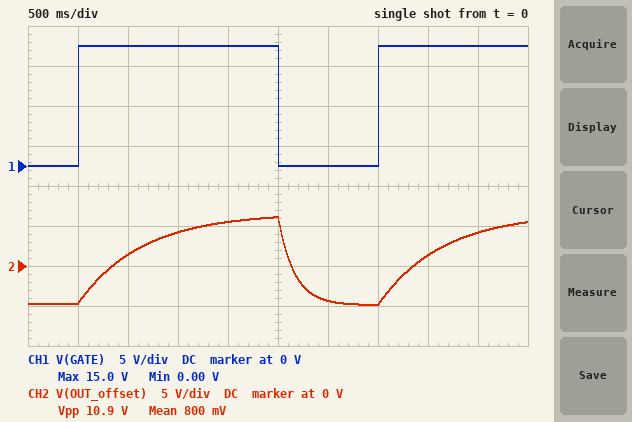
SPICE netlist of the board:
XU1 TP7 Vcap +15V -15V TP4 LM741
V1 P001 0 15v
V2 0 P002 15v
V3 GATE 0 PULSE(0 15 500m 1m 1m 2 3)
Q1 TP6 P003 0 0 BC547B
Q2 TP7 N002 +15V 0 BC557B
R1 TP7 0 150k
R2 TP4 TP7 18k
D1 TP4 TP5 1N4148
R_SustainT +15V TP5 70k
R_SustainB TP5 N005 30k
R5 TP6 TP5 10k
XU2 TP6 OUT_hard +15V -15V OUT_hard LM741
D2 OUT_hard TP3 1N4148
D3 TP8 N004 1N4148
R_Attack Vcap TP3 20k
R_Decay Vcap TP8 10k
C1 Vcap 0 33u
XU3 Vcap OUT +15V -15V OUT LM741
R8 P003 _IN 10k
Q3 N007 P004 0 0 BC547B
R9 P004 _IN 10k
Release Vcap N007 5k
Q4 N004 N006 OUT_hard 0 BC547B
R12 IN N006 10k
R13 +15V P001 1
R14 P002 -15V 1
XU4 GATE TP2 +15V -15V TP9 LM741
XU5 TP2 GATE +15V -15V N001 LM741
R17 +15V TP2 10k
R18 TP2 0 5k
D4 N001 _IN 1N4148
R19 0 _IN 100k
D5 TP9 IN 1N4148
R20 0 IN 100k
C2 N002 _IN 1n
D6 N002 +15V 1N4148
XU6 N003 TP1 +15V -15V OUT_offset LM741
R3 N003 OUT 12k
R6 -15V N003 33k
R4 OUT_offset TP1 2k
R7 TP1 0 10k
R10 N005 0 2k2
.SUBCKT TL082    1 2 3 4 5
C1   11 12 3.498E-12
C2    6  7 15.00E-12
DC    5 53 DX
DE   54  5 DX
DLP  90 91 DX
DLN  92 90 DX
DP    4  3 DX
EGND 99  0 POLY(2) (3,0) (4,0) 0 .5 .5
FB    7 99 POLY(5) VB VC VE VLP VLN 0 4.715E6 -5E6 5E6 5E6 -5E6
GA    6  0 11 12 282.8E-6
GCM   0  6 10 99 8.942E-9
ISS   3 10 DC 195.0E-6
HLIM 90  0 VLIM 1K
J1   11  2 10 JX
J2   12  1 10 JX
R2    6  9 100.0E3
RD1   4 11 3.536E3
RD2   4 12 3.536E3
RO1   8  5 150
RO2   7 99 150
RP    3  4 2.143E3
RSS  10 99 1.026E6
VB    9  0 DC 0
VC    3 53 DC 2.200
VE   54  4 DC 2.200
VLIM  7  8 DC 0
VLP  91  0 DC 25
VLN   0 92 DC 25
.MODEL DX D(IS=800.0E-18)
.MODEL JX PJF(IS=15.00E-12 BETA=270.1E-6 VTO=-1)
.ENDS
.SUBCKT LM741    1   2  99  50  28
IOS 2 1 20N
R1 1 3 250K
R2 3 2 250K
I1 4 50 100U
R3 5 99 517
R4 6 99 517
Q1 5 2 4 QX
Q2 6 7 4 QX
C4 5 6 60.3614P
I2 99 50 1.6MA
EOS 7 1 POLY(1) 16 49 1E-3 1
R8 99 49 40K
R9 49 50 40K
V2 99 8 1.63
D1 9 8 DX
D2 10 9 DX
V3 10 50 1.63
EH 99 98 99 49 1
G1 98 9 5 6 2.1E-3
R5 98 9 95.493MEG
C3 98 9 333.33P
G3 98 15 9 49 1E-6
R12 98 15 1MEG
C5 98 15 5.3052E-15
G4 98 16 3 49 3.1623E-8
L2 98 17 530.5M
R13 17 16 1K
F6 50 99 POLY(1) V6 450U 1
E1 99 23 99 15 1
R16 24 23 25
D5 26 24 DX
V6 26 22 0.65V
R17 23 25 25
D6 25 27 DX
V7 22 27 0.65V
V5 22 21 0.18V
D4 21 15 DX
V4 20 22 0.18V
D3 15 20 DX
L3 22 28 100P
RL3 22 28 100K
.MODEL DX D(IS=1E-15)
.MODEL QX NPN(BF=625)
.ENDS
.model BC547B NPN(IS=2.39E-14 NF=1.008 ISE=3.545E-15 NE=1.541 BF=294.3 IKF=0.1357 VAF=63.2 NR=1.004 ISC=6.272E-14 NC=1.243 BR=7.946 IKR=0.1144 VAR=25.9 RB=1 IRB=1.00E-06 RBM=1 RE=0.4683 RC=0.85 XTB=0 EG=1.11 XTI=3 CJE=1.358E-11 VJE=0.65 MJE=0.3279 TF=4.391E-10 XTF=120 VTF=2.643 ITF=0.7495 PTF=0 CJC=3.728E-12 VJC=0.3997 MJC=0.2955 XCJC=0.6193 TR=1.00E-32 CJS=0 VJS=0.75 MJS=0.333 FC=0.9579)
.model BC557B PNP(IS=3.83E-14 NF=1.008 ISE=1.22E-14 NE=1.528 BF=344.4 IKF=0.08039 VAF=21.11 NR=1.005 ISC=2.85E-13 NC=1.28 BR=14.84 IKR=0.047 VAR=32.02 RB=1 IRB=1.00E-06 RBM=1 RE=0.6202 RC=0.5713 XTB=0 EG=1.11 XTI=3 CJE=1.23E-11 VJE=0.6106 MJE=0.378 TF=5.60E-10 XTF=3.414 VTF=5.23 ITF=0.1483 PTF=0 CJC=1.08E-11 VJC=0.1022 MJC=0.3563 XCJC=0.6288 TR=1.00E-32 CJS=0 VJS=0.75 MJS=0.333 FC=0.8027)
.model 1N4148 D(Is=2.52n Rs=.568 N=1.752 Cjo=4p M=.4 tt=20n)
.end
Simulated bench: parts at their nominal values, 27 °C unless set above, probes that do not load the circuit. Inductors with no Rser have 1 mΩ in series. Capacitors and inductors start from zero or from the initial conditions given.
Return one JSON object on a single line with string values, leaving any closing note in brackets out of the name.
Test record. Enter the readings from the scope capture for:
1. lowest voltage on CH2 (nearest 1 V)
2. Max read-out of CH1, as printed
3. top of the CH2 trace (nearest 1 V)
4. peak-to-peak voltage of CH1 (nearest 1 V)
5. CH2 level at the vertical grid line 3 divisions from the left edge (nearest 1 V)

{"lowest voltage on CH2": "-5 V", "Max read-out of CH1, as printed": "15.0 V", "top of the CH2 trace": "6 V", "peak-to-peak voltage of CH1": "15 V", "CH2 level at the vertical grid line 3 divisions from the left edge": "4 V"}
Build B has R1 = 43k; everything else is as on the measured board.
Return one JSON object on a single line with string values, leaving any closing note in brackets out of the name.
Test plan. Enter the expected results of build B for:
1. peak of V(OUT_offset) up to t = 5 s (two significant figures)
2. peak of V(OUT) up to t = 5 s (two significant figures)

{"peak of V(OUT_offset) up to t = 5 s": "3.8 V", "peak of V(OUT) up to t = 5 s": "9.8 V"}
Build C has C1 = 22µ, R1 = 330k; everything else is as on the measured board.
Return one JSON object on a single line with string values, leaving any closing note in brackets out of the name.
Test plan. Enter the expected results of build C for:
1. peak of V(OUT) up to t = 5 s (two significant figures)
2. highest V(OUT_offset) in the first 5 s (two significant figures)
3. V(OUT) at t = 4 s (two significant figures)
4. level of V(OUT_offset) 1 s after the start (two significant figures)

{"peak of V(OUT) up to t = 5 s": "13 V", "highest V(OUT_offset) in the first 5 s": "6.6 V", "V(OUT) at t = 4 s": "9.0 V", "level of V(OUT_offset) 1 s after the start": "3.1 V"}
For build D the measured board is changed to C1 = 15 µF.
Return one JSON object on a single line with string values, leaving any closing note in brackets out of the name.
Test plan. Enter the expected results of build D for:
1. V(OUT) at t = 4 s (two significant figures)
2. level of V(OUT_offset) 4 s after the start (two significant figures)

{"V(OUT) at t = 4 s": "11 V", "level of V(OUT_offset) 4 s after the start": "4.5 V"}
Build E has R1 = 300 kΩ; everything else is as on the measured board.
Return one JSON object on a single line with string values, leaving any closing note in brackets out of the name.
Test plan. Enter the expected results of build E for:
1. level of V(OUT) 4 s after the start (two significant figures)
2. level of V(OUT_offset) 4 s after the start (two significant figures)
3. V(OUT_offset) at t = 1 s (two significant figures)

{"level of V(OUT) 4 s after the start": "7.1 V", "level of V(OUT_offset) 4 s after the start": "1.4 V", "V(OUT_offset) at t = 1 s": "1.4 V"}
